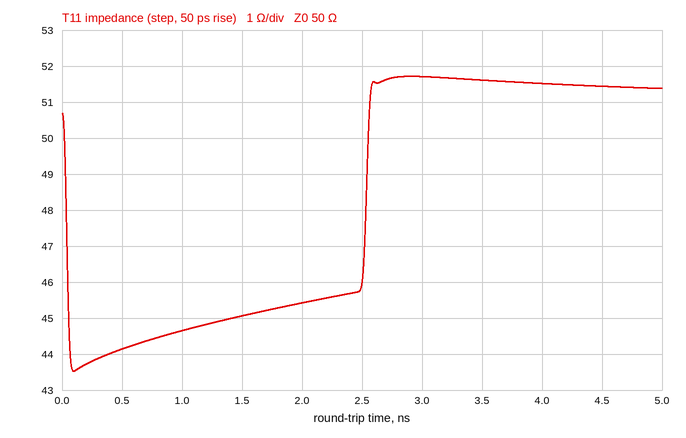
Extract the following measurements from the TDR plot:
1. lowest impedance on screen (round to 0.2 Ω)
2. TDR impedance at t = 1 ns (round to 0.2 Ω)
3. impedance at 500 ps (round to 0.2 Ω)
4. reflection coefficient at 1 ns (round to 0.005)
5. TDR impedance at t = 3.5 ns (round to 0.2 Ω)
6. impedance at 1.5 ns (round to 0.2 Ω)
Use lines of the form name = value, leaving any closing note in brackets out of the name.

lowest impedance on screen = 43.6 Ω
TDR impedance at t = 1 ns = 44.6 Ω
impedance at 500 ps = 44.2 Ω
reflection coefficient at 1 ns = -0.055
TDR impedance at t = 3.5 ns = 51.6 Ω
impedance at 1.5 ns = 45.0 Ω
